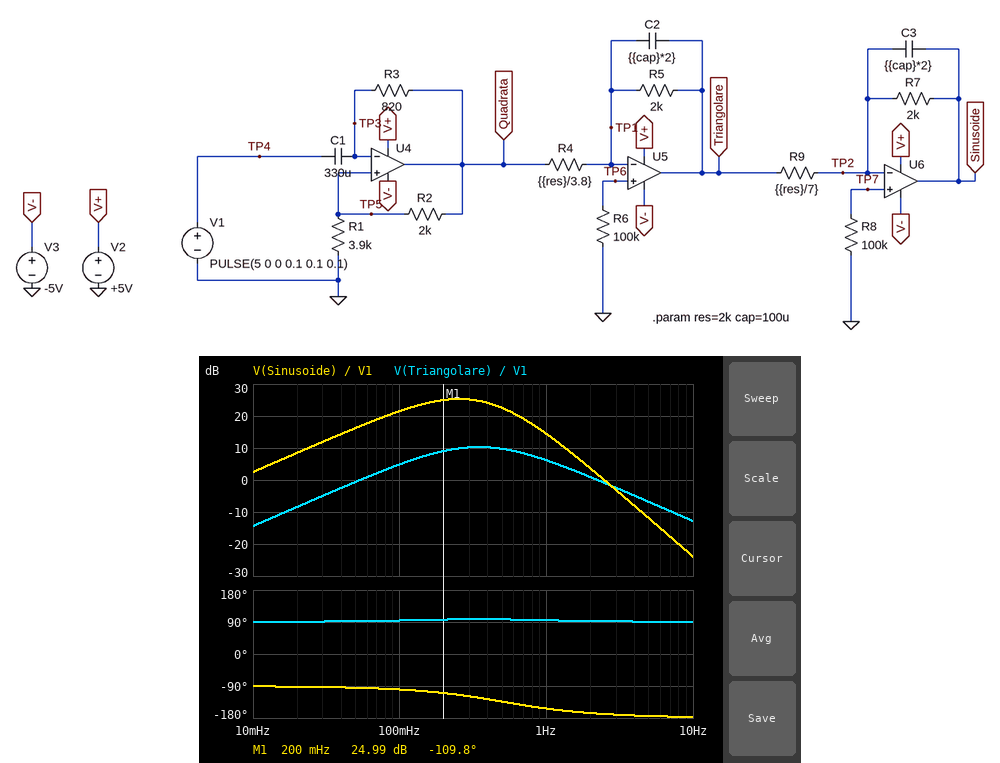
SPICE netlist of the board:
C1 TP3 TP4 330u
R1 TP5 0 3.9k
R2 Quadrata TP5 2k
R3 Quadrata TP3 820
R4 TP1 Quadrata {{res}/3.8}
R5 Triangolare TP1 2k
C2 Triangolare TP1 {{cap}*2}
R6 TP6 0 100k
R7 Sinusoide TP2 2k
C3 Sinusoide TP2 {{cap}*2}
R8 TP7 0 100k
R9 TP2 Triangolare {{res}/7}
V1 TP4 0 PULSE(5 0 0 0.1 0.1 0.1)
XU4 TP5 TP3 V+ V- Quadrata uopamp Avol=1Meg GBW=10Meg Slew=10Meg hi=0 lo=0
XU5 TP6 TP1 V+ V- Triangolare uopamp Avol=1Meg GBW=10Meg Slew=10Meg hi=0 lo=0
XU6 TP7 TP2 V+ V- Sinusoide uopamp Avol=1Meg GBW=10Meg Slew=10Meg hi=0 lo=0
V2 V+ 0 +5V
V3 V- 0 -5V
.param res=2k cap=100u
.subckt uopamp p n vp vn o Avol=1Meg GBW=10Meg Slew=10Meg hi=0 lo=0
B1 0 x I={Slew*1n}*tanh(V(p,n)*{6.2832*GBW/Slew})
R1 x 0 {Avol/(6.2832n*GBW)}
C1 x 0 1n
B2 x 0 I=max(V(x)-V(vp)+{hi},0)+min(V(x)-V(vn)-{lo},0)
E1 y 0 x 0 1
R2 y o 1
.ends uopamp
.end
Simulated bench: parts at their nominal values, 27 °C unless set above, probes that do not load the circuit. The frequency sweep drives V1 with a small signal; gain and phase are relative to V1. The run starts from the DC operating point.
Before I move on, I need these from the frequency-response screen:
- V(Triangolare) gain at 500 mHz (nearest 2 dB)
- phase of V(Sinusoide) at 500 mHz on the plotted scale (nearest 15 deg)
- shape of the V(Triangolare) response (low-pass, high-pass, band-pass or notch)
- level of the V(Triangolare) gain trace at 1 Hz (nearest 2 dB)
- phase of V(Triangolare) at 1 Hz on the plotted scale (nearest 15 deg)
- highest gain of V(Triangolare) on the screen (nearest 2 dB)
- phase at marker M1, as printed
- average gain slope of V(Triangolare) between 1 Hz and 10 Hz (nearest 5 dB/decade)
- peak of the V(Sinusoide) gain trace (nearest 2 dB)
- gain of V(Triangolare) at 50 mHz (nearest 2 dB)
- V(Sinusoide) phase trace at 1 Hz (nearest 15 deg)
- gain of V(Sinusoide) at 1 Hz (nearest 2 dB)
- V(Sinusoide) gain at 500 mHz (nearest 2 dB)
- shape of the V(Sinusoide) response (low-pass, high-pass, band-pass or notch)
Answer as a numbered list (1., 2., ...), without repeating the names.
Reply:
1. 10 dB
2. -135 deg
3. band-pass
4. 6 dB
5. 90 deg
6. 10 dB
7. -109.8 deg
8. -20 dB/decade
9. 26 dB
10. 0 dB
11. -150 deg
12. 14 dB
13. 22 dB
14. band-pass
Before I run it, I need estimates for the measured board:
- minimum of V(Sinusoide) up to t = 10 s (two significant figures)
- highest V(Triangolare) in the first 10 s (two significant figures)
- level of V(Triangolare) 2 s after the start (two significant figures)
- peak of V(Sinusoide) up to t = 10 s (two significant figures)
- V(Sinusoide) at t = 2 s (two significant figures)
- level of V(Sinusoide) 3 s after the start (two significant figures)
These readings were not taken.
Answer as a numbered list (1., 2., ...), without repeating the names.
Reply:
1. -5.0 V
2. 5.0 V
3. -5.0 V
4. 5.0 V
5. 5.0 V
6. 5.0 V
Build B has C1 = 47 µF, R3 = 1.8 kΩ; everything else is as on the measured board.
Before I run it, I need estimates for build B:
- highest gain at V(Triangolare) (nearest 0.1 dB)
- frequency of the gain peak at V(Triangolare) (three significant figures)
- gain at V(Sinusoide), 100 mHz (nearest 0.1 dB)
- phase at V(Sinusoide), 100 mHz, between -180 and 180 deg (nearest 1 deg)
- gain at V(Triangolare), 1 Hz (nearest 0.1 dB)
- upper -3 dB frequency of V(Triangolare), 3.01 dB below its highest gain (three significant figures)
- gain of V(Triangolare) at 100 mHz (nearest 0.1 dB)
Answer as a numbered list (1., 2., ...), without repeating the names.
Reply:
1. 4.5 dB
2. 620 mHz
3. 11.8 dB
4. -112 deg
5. 3.7 dB
6. 1.60 Hz
7. -4.8 dB
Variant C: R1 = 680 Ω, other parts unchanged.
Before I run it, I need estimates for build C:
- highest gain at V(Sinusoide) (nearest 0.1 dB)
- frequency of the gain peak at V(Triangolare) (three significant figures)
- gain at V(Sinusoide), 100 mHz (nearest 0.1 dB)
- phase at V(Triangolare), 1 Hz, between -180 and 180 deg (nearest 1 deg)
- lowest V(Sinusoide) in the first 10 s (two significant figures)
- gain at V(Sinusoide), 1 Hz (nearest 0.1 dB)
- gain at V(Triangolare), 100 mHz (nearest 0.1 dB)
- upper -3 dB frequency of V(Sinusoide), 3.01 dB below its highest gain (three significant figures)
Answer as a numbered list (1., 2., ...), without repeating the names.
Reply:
1. 21.4 dB
2. 830 mHz
3. 15.1 dB
4. 52 deg
5. -5.0 V
6. 17.1 dB
7. -1.5 dB
8. 849 mHz
